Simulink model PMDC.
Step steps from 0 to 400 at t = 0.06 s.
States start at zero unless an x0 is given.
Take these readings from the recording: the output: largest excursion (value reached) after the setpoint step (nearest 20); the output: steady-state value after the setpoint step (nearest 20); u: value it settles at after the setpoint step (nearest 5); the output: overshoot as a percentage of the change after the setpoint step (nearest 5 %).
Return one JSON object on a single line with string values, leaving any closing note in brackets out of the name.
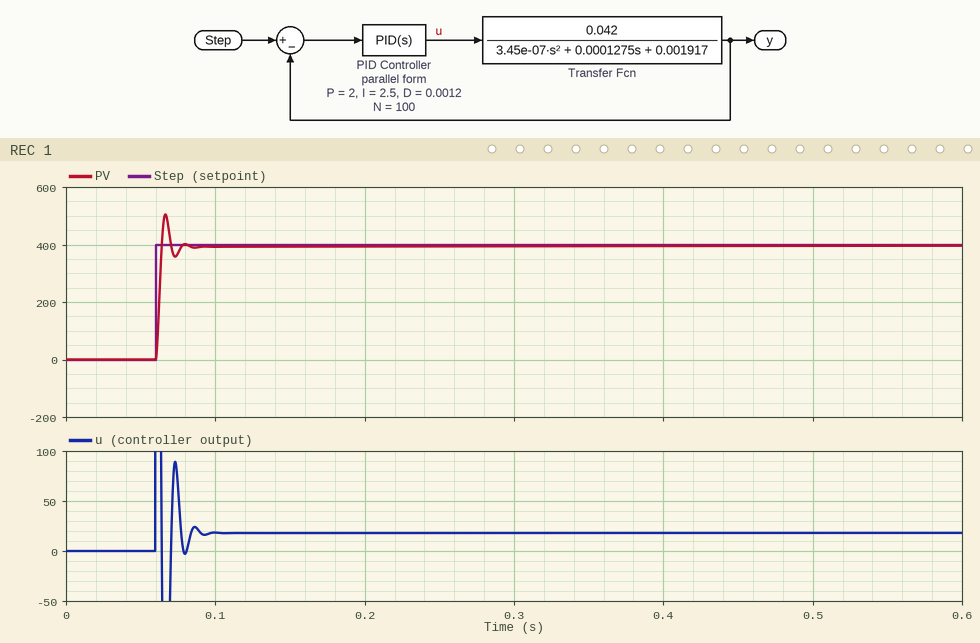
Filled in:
{"the output: largest excursion (value reached) after the setpoint step": "500", "the output: steady-state value after the setpoint step": "400", "u: value it settles at after the setpoint step": "20", "the output: overshoot as a percentage of the change after the setpoint step": "25 %"}
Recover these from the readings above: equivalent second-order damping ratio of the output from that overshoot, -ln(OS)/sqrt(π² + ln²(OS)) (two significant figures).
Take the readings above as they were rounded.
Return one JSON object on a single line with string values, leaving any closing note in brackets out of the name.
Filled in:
{"equivalent second-order damping ratio of the output from that overshoot, -ln(OS)/sqrt(π² + ln²(OS))": "0.40"}
